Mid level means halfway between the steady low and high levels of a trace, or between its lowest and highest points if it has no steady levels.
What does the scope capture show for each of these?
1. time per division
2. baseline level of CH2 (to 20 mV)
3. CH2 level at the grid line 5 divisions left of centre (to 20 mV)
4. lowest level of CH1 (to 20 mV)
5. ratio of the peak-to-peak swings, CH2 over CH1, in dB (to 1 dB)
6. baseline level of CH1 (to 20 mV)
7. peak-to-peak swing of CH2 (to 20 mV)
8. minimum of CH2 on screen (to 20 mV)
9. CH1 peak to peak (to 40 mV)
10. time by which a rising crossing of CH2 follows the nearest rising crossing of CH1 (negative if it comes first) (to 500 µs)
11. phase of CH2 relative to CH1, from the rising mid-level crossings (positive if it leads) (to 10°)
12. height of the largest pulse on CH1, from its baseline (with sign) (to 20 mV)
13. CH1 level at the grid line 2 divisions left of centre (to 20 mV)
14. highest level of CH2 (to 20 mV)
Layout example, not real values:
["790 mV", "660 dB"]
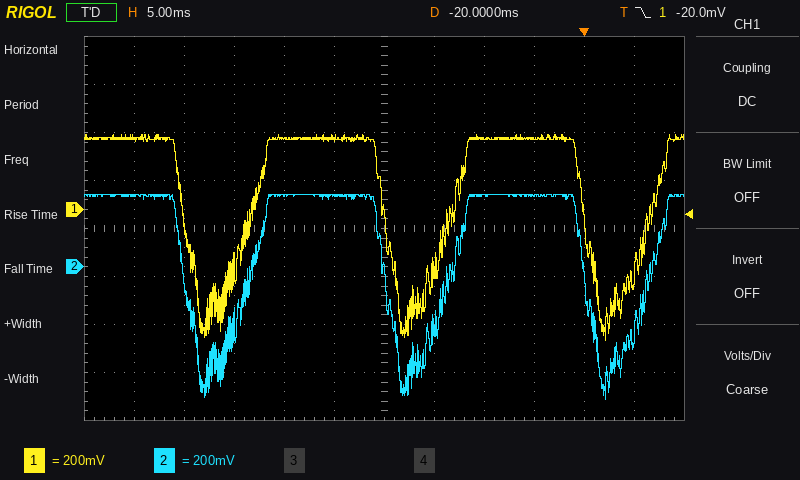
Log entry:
["5 ms", "300 mV", "300 mV", "-540 mV", "0 dB", "300 mV", "860 mV", "-560 mV", "840 mV", "0.0 ms", "0°", "-840 mV", "300 mV", "300 mV"]
